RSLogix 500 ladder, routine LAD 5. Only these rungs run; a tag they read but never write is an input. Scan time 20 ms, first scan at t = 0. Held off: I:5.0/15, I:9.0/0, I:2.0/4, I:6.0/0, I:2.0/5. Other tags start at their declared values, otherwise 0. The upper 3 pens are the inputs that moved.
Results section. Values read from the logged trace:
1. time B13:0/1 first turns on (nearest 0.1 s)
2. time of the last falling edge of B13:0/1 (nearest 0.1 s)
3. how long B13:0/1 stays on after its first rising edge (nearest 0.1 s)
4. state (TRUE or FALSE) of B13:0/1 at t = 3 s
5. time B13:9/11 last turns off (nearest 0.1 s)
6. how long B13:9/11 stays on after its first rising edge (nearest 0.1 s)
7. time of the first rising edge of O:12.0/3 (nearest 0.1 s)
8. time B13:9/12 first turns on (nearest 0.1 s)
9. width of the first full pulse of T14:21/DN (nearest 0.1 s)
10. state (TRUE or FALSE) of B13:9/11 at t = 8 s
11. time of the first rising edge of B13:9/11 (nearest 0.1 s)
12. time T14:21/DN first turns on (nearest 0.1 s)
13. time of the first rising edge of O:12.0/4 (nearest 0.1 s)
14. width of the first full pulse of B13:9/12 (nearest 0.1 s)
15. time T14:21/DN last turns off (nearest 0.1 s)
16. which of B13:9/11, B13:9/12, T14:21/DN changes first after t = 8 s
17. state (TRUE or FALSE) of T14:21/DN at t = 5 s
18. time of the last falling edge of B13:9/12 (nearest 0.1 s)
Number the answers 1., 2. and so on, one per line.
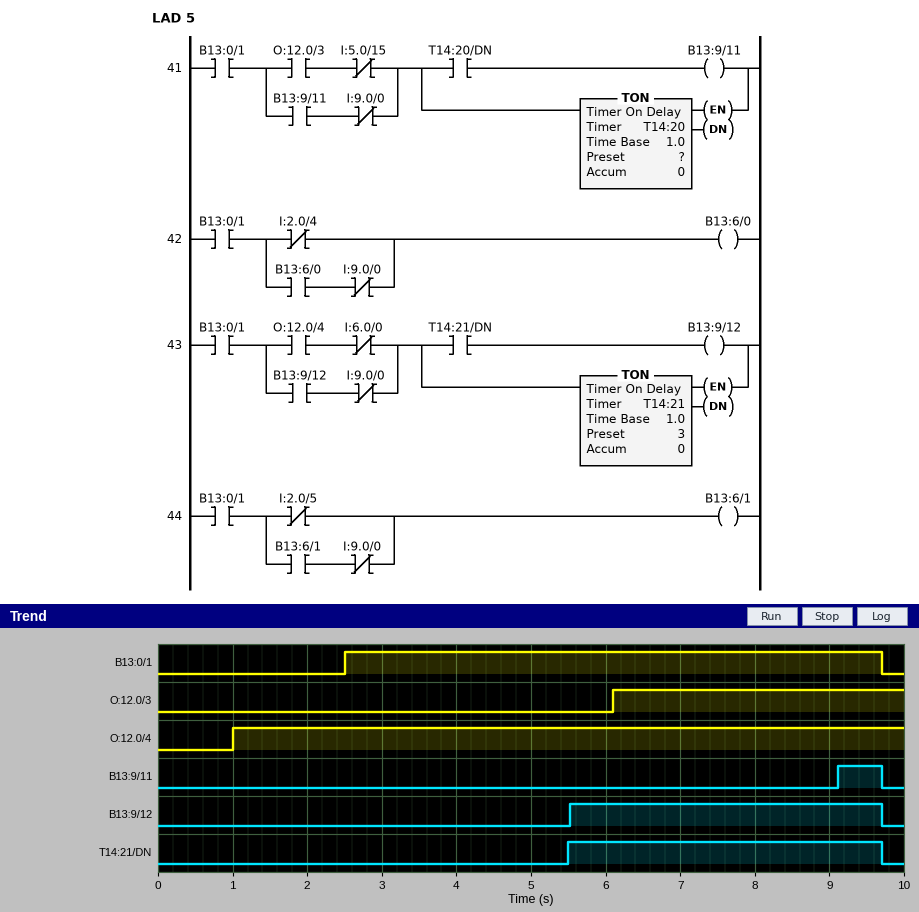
1. 2.5 s
2. 9.7 s
3. 7.2 s
4. TRUE
5. 9.7 s
6. 0.6 s
7. 6.1 s
8. 5.5 s
9. 4.2 s
10. FALSE
11. 9.1 s
12. 5.5 s
13. 1.0 s
14. 4.2 s
15. 9.7 s
16. B13:9/11
17. FALSE
18. 9.7 s
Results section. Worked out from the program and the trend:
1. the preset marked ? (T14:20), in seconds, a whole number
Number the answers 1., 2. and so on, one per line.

1. 3 s
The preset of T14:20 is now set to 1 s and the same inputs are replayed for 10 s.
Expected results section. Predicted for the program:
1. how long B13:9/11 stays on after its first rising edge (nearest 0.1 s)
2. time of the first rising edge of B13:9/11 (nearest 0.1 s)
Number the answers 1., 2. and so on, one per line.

1. 2.6 s
2. 7.1 s
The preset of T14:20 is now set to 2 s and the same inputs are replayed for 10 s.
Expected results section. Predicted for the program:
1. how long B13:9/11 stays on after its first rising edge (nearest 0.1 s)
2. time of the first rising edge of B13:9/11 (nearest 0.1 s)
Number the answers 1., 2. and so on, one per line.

1. 1.6 s
2. 8.1 s
